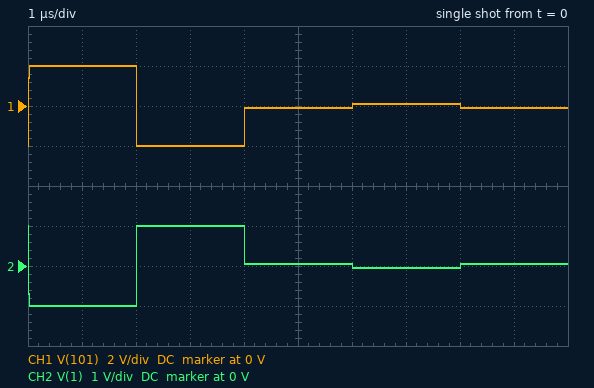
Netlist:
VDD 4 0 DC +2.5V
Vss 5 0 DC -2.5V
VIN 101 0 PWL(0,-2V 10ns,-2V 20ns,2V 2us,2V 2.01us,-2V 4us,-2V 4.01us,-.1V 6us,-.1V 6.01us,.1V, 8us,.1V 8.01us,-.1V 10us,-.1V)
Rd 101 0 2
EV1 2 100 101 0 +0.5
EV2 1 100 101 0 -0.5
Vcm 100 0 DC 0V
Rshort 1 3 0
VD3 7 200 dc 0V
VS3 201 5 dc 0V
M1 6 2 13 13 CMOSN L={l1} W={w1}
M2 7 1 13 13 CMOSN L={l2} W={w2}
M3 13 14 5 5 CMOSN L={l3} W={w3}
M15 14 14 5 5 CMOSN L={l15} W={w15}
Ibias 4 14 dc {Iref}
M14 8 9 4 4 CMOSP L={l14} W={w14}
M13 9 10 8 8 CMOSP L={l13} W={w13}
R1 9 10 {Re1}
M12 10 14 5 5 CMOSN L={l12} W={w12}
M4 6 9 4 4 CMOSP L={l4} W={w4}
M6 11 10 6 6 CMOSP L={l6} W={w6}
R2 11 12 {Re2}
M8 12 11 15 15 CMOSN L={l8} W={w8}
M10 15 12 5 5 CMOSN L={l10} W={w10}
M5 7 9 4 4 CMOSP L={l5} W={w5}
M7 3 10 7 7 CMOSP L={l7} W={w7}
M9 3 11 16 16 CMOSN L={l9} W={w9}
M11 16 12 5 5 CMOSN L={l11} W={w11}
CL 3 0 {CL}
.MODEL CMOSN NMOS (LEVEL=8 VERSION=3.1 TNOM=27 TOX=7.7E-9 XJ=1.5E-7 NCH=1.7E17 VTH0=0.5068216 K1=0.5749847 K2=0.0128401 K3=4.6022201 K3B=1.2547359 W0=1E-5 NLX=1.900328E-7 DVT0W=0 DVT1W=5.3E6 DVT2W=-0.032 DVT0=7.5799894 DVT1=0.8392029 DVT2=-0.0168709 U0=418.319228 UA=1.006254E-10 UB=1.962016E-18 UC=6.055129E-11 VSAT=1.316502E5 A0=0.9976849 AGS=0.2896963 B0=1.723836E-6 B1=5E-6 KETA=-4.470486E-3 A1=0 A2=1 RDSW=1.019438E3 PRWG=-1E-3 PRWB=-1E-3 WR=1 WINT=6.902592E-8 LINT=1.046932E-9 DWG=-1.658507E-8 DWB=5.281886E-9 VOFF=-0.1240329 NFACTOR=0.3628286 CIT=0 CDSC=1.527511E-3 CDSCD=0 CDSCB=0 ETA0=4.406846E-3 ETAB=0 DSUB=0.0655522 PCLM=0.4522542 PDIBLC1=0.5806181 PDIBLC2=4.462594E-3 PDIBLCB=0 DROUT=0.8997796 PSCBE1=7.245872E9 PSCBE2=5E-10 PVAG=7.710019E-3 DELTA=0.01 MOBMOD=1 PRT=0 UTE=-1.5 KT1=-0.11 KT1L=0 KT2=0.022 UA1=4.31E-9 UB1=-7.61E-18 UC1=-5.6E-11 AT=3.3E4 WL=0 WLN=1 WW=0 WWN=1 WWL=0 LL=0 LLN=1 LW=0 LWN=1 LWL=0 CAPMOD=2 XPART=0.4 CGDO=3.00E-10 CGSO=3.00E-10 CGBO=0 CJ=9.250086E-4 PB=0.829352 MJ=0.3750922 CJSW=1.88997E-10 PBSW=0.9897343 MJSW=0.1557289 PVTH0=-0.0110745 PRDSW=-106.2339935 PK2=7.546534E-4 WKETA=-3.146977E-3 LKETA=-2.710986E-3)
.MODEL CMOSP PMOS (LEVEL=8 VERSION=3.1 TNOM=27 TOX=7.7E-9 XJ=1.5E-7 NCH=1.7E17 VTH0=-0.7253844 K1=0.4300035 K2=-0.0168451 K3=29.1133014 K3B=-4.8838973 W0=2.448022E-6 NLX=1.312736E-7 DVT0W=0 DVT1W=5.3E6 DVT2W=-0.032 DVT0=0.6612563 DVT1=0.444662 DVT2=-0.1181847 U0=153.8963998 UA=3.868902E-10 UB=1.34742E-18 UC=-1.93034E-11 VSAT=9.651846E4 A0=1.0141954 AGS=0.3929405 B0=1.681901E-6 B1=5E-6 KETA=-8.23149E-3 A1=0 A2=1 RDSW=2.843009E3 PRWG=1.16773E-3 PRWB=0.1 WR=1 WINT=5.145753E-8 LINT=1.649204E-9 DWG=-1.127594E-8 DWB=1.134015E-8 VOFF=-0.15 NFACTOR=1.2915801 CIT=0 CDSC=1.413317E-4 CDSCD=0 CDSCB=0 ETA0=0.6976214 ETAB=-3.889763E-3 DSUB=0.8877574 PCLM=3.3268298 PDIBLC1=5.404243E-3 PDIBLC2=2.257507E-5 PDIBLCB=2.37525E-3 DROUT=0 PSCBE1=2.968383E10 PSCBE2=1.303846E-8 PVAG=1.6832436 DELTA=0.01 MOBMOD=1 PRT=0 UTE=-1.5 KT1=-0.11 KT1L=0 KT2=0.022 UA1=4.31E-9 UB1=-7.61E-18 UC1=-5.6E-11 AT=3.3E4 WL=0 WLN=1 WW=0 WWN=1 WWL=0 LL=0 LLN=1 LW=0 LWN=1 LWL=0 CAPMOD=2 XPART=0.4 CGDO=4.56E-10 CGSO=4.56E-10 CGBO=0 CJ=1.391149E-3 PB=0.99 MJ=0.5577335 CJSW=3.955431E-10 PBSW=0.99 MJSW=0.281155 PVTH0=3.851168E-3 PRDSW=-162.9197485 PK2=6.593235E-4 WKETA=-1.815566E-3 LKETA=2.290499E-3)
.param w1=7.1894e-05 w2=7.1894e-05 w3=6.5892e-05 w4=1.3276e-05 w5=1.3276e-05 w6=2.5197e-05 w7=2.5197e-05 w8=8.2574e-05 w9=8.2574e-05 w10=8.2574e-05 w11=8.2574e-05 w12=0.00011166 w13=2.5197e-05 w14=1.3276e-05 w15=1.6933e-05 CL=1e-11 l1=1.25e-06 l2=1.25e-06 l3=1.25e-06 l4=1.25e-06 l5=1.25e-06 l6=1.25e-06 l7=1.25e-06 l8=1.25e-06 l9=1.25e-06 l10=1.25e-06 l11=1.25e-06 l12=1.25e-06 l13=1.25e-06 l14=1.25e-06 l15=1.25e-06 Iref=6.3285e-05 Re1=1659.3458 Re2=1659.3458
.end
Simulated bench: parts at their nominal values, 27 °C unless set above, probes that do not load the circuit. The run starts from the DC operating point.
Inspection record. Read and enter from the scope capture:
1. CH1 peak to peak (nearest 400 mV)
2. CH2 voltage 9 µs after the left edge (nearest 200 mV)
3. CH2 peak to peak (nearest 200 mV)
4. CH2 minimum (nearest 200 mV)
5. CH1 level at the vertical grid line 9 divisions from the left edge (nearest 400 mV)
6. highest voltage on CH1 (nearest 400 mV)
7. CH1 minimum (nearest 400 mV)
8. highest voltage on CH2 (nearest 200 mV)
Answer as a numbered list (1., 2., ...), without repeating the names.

1. 4.0 V
2. 0 V
3. 2.0 V
4. -1.0 V
5. 0 V
6. 2.0 V
7. -2.0 V
8. 1.0 V
